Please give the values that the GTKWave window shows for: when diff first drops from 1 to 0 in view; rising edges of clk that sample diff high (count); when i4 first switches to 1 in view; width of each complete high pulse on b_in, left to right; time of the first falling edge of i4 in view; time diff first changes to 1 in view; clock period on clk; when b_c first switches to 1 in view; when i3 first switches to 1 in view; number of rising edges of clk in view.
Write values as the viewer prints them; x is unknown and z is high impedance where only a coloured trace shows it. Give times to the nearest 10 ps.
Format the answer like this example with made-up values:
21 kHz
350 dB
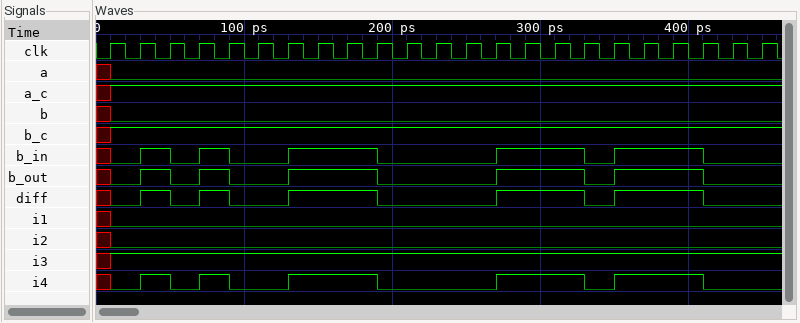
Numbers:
50 ps
11
30 ps
20 ps, 20 ps, 60 ps, 60 ps, 60 ps
50 ps
30 ps
20 ps
10 ps
10 ps
23
